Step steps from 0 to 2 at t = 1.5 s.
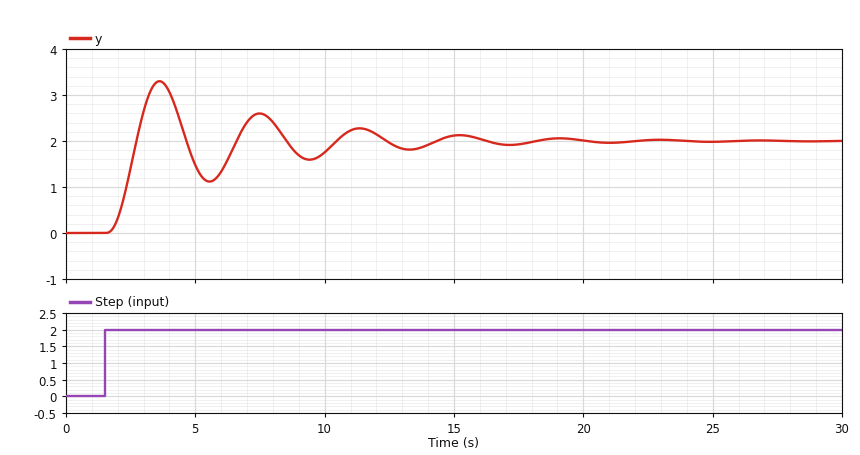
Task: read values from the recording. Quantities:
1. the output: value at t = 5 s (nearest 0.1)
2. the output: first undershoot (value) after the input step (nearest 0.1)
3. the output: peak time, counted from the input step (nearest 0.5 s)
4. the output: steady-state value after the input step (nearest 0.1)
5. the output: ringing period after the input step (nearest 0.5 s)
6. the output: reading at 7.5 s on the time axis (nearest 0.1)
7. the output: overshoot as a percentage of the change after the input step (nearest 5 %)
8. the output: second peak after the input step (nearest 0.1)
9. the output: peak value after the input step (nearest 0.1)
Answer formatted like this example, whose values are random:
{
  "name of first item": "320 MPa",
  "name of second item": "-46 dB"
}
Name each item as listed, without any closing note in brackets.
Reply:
{
  "the output: value at t = 5 s": "1.5",
  "the output: first undershoot (value) after the input step": "1.1",
  "the output: peak time, counted from the input step": "2.0 s",
  "the output: steady-state value after the input step": "2.0",
  "the output: ringing period after the input step": "4.0 s",
  "the output: reading at 7.5 s on the time axis": "2.6",
  "the output: overshoot as a percentage of the change after the input step": "65 %",
  "the output: second peak after the input step": "2.6",
  "the output: peak value after the input step": "3.3"
}
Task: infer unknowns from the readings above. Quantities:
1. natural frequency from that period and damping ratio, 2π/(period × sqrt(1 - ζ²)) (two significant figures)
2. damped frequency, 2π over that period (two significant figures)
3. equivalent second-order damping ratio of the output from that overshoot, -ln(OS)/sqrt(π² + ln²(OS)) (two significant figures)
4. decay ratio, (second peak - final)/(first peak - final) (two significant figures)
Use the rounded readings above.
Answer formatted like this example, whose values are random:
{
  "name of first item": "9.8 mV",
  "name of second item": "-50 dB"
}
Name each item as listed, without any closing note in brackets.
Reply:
{
  "natural frequency from that period and damping ratio, 2π/(period × sqrt(1 - ζ²))": "1.6 rad/s",
  "damped frequency, 2π over that period": "1.6 rad/s",
  "equivalent second-order damping ratio of the output from that overshoot, -ln(OS)/sqrt(π² + ln²(OS))": "0.14",
  "decay ratio, (second peak - final)/(first peak - final)": "0.46"
}
